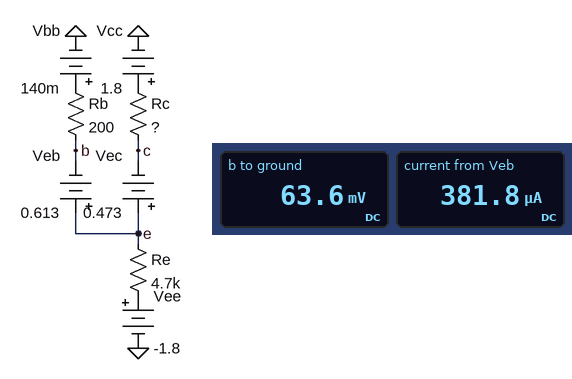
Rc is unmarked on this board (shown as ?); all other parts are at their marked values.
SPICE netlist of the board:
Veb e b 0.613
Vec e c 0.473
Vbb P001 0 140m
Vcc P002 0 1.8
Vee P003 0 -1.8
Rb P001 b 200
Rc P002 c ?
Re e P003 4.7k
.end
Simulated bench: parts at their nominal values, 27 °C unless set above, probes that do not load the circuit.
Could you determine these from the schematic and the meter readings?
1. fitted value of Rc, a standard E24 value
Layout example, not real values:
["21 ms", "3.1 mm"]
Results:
["11 kΩ"]
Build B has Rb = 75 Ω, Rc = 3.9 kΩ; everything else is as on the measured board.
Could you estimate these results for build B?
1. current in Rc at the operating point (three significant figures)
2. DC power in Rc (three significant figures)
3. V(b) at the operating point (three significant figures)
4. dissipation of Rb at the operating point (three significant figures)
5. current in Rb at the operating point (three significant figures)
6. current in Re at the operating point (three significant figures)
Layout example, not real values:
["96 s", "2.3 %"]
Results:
["393 µA", "601 µW", "129 mV", "1.65 µW", "148 µA", "541 µA"]
